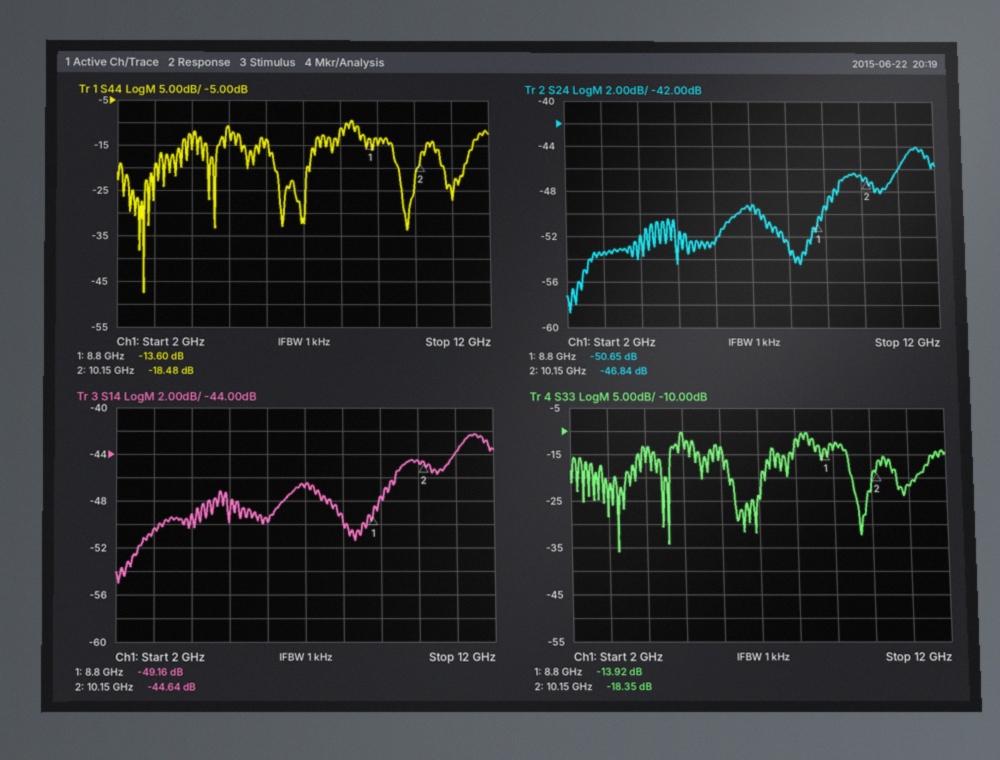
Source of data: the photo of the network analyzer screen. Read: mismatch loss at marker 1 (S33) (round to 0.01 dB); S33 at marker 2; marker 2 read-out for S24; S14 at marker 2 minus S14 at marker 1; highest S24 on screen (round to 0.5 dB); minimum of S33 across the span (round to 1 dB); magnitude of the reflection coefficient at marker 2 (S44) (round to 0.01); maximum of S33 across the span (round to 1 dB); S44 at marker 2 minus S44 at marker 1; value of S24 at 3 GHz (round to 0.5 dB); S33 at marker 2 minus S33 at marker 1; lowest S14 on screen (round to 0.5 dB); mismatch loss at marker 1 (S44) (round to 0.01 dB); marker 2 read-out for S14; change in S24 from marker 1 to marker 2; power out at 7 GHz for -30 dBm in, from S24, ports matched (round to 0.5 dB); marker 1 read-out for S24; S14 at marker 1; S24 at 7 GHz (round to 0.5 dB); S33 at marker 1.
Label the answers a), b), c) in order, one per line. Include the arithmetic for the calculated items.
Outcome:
a) −10 log10(1 − 10^(-13.92/10)) ≈ 0.18 dB
b) -18.35 dB
c) -46.84 dB
d) -44.64 − (-49.16) = 4.52 dB
e) -44.0 dB
f) -36 dB
g) 10^(-18.48/20) ≈ 0.12
h) -10 dB
i) -18.48 − (-13.6) = -4.88 dB
j) -53.5 dB
k) -18.35 − (-13.92) = -4.43 dB
l) -55.0 dB
m) −10 log10(1 − 10^(-13.6/10)) ≈ 0.19 dB
n) -44.64 dB
o) -46.84 − (-50.65) = 3.81 dB
p) -30 dBm + (-49.5 dB) = -79.5 dBm
q) -50.65 dB
r) -49.16 dB
s) -49.5 dB
t) -13.92 dB
